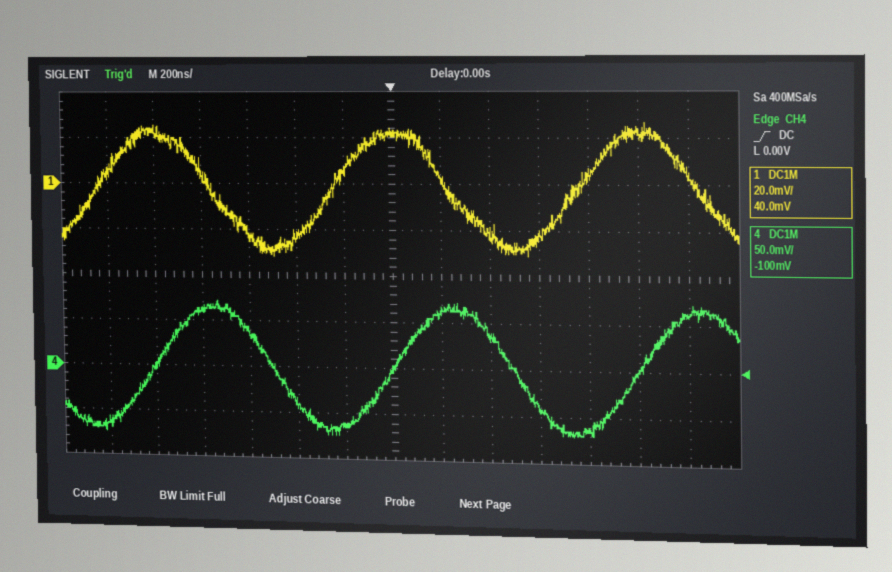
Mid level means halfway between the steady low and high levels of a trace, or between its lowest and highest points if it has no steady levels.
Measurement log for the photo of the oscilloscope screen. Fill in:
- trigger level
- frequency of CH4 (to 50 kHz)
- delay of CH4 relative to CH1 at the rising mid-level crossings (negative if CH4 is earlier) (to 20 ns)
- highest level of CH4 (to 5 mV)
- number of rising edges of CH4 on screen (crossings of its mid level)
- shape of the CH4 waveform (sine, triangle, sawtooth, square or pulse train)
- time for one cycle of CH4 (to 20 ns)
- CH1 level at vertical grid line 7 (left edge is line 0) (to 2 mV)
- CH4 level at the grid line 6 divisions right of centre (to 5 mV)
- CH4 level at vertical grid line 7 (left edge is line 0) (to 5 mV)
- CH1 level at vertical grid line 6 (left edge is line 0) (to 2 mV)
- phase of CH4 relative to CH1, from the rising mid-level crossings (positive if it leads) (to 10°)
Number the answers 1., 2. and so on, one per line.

1. 0.00 V
2. 1.00 MHz
3. +240 ns
4. 70 mV
5. 3
6. sine
7. 1.00 µs
8. 22 mV
9. 60 mV
10. 0 mV
11. 6 mV
12. -90°
